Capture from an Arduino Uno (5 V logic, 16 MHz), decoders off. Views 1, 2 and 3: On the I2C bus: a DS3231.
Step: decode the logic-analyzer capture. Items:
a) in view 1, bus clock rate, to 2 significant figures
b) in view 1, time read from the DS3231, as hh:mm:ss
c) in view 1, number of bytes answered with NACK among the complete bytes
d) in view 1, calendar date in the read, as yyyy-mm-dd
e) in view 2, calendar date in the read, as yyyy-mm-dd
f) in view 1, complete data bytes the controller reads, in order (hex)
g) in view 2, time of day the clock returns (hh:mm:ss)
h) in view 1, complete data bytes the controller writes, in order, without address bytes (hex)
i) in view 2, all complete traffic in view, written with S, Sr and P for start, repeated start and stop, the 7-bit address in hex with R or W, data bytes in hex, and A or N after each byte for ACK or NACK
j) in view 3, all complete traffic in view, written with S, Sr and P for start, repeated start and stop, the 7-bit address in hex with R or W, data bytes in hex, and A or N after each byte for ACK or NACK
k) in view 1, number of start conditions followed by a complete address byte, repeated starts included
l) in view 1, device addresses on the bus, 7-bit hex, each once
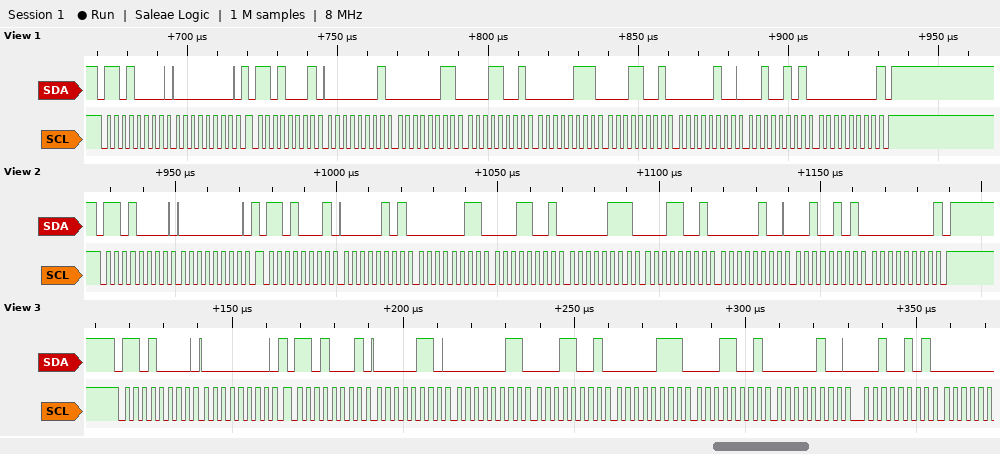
400 kHz
19:03:01
1
2025-04-19
2025-04-19
01 03 19 07 19 04 25 00
19:03:05
00
S 68W A 00 A Sr 68R A 05 A 03 A 19 A 07 A 19 A 04 A 25 A 00 N P
S 68W A 00 A Sr 68R A 06 A 03 A 19 A 07 A 19 A 04 A 25 A
2
0x68
